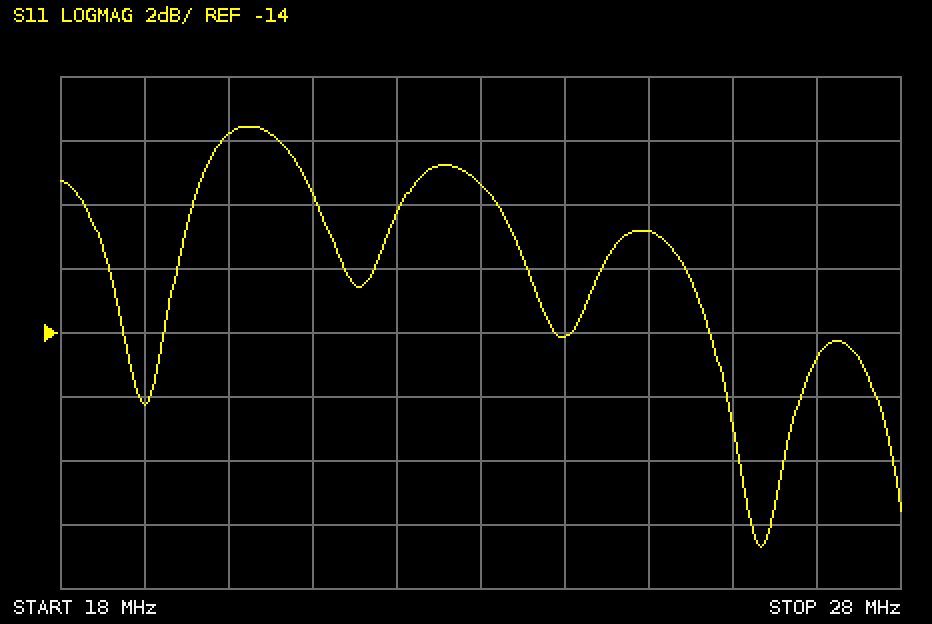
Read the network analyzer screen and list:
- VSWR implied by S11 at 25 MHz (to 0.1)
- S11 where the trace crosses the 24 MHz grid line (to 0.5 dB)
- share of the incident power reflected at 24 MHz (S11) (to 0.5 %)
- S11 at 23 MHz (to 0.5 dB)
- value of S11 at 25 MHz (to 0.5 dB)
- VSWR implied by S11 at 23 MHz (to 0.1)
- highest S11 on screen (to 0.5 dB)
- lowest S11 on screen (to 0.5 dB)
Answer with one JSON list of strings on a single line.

["1.8", "-14.0 dB", "4.0 %", "-9.5 dB", "-11.0 dB", "2.0", "-7.5 dB", "-20.5 dB"]
